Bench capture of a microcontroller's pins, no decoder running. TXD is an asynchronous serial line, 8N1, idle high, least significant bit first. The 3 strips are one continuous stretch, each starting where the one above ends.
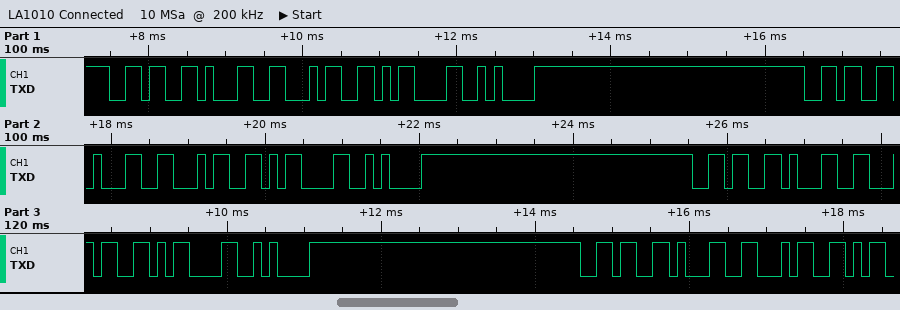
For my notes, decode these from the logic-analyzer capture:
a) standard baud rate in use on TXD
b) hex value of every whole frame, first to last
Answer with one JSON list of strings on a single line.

["9600 baud", "0x36 0x31 0x34 0x0D 0x0A 0x36 0x31 0x34 0x0D 0x0A 0x36 0x31 0x34 0x0D 0x0A 0x36 0x31 0x34"]
